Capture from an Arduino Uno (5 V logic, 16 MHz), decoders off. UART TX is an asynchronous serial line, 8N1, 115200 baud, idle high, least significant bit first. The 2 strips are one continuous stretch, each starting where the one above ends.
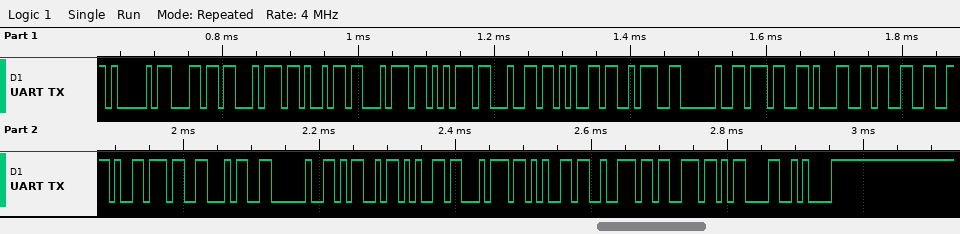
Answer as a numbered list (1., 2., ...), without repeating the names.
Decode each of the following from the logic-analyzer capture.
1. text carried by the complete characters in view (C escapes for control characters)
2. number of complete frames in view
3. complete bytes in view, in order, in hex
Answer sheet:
1. "Altitude: 713.74 Meters\r\n"
2. 25
3. 41 6C 74 69 74 75 64 65 3A 20 37 31 33 2E 37 34 20 4D 65 74 65 72 73 0D 0A
